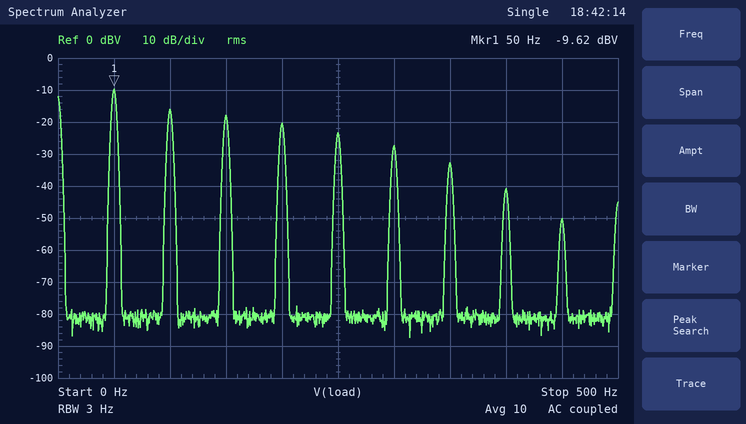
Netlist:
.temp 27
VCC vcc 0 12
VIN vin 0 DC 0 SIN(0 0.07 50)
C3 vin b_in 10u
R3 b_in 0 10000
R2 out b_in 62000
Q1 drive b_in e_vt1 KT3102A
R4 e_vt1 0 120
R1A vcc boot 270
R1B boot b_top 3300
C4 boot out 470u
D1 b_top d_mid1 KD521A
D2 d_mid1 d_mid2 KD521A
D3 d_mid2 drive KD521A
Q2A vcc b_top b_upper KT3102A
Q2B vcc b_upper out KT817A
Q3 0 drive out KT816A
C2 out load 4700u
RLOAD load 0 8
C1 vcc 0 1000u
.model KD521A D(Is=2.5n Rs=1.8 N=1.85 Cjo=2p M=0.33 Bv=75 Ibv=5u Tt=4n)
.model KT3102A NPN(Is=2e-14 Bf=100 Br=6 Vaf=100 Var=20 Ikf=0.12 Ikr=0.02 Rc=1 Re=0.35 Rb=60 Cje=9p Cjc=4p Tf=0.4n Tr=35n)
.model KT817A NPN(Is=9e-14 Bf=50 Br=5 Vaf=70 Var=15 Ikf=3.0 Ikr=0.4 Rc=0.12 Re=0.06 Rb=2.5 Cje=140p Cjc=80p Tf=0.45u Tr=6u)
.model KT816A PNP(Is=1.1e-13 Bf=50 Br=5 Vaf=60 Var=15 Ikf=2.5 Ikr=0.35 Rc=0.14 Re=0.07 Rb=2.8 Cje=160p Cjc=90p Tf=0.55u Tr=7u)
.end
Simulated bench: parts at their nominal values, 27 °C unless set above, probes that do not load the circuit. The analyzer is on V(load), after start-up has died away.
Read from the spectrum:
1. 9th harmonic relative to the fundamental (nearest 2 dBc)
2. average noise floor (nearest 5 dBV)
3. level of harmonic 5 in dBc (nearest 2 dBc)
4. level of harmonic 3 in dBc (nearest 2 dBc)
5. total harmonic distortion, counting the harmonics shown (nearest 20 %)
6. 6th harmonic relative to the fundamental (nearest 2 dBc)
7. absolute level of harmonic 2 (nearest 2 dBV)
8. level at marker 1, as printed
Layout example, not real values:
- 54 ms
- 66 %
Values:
- -40 dBc
- -80 dBV
- -14 dBc
- -8 dBc
- 80 %
- -18 dBc
- -16 dBV
- -9.62 dBV
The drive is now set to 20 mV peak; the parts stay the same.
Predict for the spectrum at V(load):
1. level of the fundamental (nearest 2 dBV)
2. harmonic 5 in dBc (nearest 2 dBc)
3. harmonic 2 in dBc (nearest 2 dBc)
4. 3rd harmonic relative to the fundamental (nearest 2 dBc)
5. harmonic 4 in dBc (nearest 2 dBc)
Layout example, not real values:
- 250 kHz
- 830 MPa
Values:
- -24 dBV
- -42 dBc
- -18 dBc
- -26 dBc
- -34 dBc
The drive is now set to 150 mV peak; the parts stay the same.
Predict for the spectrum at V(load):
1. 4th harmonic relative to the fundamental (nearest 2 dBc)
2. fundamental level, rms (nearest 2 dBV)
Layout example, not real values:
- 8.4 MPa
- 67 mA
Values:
- -10 dBc
- -2 dBV
